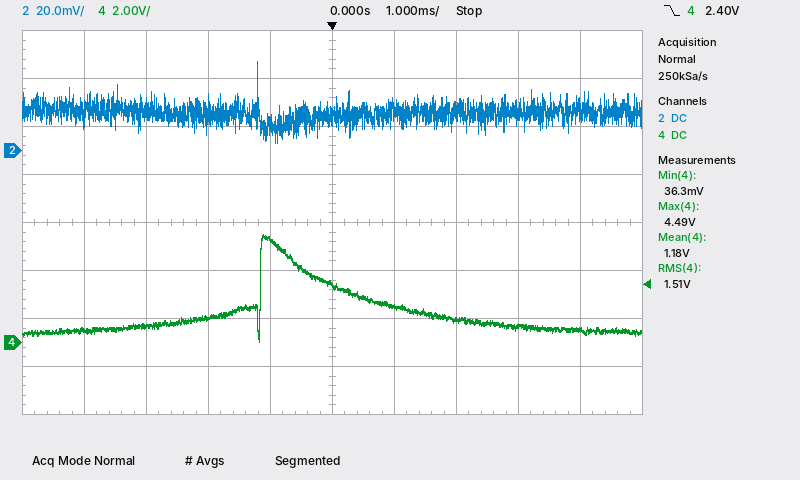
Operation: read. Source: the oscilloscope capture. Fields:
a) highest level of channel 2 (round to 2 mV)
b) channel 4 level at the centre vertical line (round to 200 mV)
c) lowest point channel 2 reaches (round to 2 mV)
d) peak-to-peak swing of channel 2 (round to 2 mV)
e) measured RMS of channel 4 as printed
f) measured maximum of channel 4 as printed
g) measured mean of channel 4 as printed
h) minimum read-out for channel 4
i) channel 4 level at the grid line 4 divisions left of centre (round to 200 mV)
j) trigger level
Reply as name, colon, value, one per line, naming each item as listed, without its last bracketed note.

highest level of channel 2: 38 mV
channel 4 level at the centre vertical line: 2.4 V
lowest point channel 2 reaches: 4 mV
peak-to-peak swing of channel 2: 34 mV
measured RMS of channel 4 as printed: 1.51 V
measured maximum of channel 4 as printed: 4.49 V
measured mean of channel 4 as printed: 1.18 V
minimum read-out for channel 4: 36.3 mV
channel 4 level at the grid line 4 divisions left of centre: 600 mV
trigger level: 2.40 V
